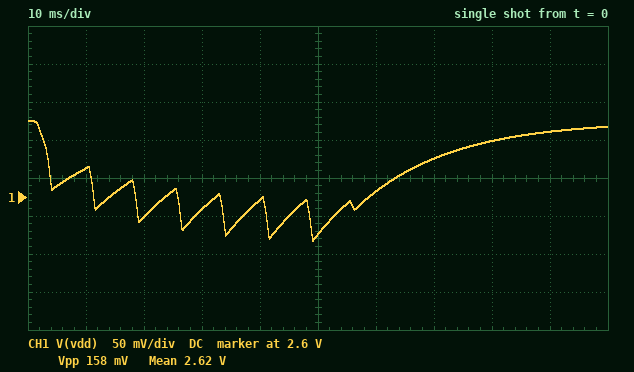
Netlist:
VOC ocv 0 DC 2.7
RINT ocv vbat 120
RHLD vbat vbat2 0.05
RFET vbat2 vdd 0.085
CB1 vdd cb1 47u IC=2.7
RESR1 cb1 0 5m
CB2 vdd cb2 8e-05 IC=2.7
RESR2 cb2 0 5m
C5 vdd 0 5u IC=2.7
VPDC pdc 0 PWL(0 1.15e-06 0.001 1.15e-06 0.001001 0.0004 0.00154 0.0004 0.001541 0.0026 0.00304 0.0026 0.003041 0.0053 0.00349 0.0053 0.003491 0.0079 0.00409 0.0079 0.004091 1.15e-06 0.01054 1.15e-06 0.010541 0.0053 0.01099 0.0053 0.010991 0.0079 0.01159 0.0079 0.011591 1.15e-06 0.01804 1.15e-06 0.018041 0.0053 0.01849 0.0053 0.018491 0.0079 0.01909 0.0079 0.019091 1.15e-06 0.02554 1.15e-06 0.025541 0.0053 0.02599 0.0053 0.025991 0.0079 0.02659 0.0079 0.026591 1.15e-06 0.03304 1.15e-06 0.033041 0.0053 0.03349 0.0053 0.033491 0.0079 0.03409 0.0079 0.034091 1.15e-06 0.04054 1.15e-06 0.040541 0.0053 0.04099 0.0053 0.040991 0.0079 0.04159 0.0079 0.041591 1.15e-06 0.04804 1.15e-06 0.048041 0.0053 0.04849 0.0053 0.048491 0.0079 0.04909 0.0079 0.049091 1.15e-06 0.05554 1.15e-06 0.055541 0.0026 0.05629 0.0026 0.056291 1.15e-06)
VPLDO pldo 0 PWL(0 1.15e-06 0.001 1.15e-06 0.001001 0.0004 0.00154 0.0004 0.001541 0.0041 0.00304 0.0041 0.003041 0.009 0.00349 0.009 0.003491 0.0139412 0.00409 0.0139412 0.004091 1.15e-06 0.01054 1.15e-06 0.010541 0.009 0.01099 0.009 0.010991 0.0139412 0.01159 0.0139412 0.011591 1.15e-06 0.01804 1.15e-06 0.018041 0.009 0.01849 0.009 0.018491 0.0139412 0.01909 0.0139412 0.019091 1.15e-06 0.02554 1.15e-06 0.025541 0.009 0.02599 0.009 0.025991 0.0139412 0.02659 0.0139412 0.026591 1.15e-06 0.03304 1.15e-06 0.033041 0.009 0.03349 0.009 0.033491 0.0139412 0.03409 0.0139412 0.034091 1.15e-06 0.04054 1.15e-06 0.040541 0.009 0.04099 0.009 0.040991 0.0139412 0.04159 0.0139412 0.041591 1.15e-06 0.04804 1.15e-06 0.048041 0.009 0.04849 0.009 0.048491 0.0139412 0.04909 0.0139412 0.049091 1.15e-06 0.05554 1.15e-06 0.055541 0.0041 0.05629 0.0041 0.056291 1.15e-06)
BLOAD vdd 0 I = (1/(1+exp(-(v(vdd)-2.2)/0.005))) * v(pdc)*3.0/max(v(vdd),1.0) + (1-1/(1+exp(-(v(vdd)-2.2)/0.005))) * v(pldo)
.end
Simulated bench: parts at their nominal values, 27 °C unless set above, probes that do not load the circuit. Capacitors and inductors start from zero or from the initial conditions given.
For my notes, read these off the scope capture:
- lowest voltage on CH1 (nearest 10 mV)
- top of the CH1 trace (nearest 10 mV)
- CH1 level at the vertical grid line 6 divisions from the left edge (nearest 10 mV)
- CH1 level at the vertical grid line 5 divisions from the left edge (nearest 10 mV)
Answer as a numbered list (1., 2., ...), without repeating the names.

1. 2.54 V
2. 2.70 V
3. 2.61 V
4. 2.55 V
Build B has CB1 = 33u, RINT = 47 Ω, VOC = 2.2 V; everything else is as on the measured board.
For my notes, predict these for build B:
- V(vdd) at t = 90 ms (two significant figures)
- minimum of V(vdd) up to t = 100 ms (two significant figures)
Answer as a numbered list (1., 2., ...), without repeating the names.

1. 2.2 V
2. 2.1 V
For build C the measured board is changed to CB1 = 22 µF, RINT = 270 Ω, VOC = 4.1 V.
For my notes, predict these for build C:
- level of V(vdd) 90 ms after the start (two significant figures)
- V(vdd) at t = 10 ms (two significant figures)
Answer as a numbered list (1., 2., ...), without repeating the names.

1. 4.0 V
2. 3.0 V
